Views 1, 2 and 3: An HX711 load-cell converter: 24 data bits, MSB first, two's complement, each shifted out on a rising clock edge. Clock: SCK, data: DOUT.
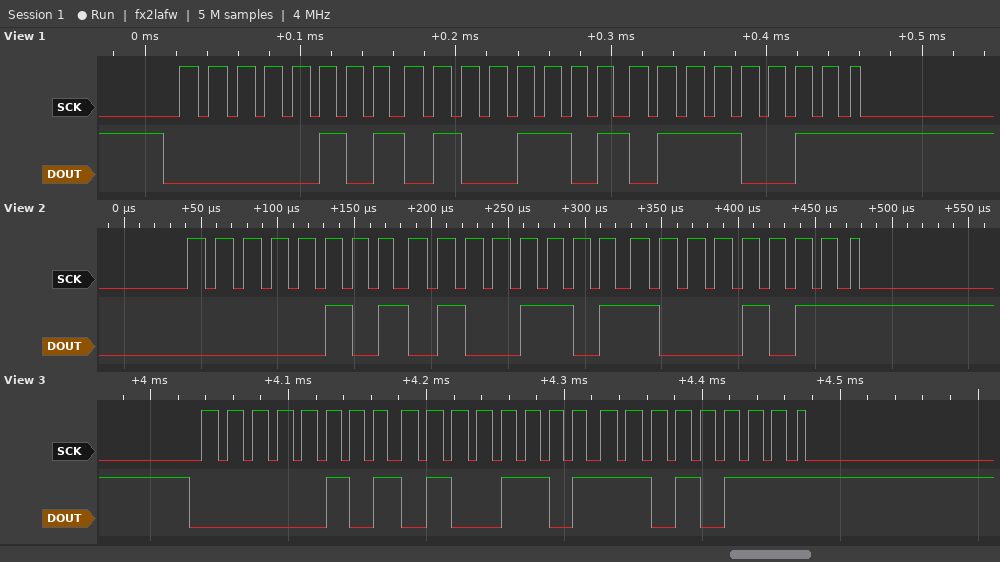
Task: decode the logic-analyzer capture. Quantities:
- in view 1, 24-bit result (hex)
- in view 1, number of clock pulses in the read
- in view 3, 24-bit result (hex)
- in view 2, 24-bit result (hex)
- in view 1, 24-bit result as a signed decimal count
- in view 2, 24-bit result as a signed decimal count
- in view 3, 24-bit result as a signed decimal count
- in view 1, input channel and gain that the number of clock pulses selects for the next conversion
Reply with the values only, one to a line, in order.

0x054D73
25
0x054DD7
0x054D8B
347507
347531
347607
channel A, gain 128
